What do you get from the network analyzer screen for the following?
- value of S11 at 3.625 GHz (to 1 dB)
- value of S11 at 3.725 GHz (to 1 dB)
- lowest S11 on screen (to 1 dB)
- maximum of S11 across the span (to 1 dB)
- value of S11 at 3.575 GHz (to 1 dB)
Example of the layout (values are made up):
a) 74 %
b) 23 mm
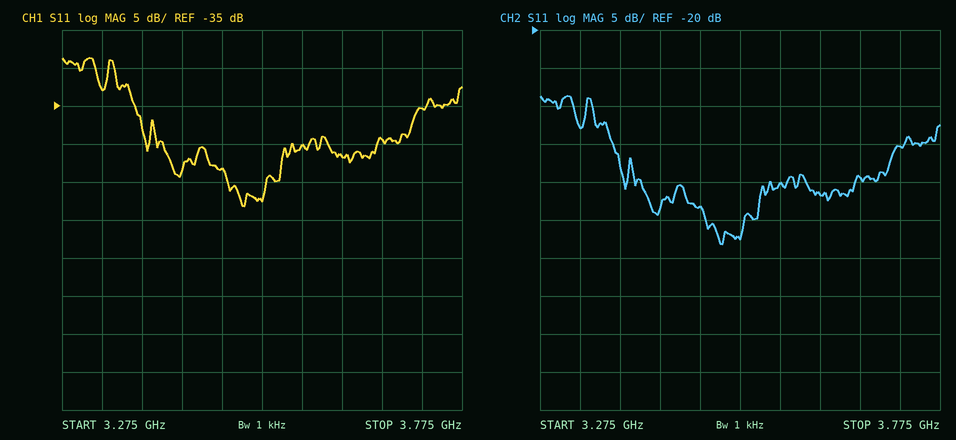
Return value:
a) -42 dB
b) -35 dB
c) -48 dB
d) -29 dB
e) -40 dB
